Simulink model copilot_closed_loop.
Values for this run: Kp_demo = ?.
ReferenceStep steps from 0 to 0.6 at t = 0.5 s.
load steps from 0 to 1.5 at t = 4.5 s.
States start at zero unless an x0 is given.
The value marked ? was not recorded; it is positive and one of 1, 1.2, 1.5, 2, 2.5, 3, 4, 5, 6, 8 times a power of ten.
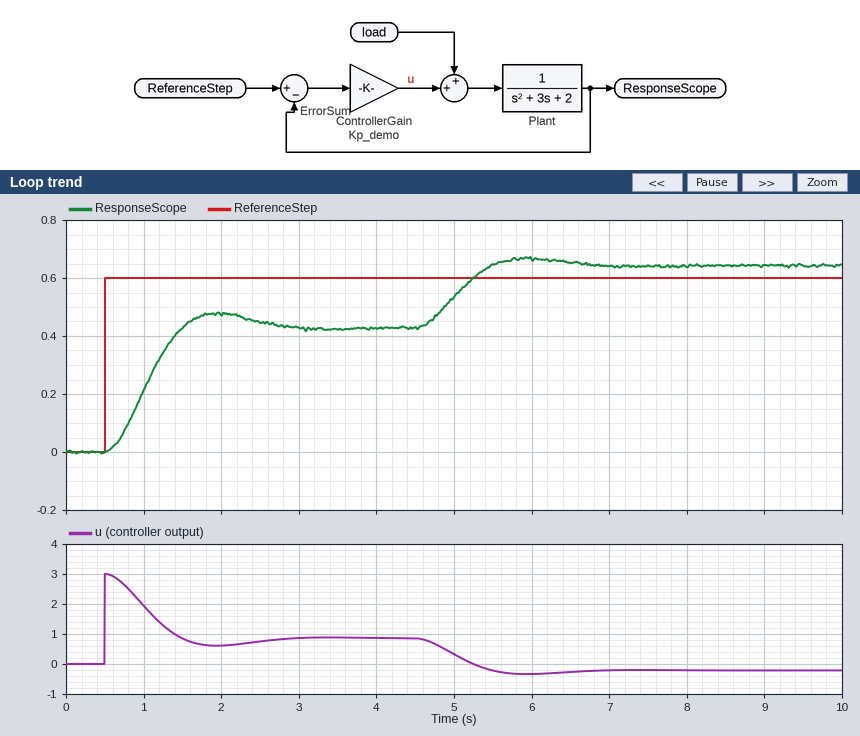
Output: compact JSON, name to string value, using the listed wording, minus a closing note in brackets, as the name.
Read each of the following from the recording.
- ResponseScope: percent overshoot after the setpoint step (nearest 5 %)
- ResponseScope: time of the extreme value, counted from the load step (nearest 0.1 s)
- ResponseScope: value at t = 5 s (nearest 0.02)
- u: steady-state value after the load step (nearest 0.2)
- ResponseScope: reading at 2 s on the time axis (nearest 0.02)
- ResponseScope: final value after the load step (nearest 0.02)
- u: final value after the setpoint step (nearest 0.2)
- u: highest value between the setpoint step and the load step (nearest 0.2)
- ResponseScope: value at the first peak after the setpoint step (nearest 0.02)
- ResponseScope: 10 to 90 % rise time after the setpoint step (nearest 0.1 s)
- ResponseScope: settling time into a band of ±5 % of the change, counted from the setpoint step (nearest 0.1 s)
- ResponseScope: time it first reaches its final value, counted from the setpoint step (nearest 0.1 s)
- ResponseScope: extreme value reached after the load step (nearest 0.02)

{"ResponseScope: percent overshoot after the setpoint step": "10 %", "ResponseScope: time of the extreme value, counted from the load step": "1.4 s", "ResponseScope: value at t = 5 s": "0.54", "u: steady-state value after the load step": "-0.2", "ResponseScope: reading at 2 s on the time axis": "0.48", "ResponseScope: final value after the load step": "0.64", "u: final value after the setpoint step": "0.8", "u: highest value between the setpoint step and the load step": "3.0", "ResponseScope: value at the first peak after the setpoint step": "0.48", "ResponseScope: 10 to 90 % rise time after the setpoint step": "0.7 s", "ResponseScope: settling time into a band of ±5 % of the change, counted from the setpoint step": "2.0 s", "ResponseScope: time it first reaches its final value, counted from the setpoint step": "1.0 s", "ResponseScope: extreme value reached after the load step": "0.66"}
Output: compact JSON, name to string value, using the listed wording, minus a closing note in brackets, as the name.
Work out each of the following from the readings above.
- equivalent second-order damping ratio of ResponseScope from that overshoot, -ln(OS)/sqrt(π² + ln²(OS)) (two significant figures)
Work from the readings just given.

{"equivalent second-order damping ratio of ResponseScope from that overshoot, -ln(OS)/sqrt(π² + ln²(OS))": "0.59"}
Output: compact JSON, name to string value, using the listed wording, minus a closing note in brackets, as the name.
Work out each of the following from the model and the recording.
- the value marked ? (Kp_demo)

{"the value marked ?": "5"}
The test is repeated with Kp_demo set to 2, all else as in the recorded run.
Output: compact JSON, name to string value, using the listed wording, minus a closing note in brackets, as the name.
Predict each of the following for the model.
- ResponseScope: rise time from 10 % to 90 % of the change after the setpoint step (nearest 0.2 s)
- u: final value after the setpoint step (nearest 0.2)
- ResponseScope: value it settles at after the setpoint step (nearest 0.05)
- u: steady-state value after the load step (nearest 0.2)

{"ResponseScope: rise time from 10 % to 90 % of the change after the setpoint step": "1.2 s", "u: final value after the setpoint step": "0.6", "ResponseScope: value it settles at after the setpoint step": "0.30", "u: steady-state value after the load step": "-0.2"}
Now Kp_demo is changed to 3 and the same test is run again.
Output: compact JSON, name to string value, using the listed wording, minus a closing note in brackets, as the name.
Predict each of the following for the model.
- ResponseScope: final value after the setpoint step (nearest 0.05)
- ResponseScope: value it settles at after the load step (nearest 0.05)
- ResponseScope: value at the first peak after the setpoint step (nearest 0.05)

{"ResponseScope: final value after the setpoint step": "0.35", "ResponseScope: value it settles at after the load step": "0.65", "ResponseScope: value at the first peak after the setpoint step": "0.40"}
